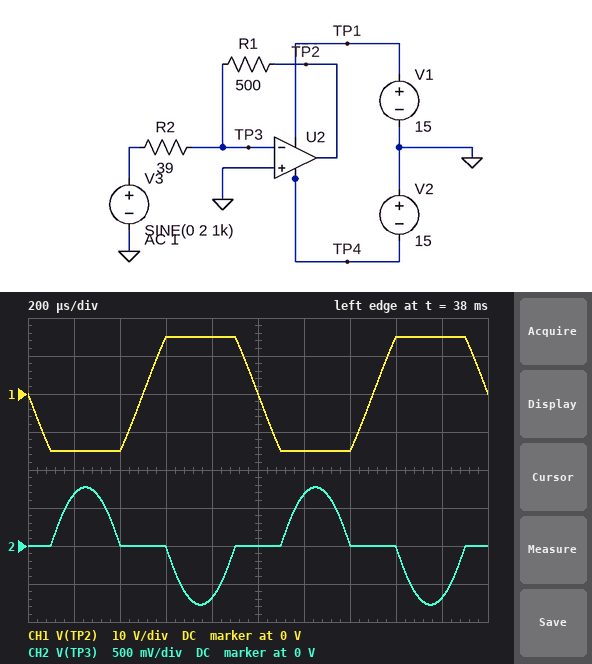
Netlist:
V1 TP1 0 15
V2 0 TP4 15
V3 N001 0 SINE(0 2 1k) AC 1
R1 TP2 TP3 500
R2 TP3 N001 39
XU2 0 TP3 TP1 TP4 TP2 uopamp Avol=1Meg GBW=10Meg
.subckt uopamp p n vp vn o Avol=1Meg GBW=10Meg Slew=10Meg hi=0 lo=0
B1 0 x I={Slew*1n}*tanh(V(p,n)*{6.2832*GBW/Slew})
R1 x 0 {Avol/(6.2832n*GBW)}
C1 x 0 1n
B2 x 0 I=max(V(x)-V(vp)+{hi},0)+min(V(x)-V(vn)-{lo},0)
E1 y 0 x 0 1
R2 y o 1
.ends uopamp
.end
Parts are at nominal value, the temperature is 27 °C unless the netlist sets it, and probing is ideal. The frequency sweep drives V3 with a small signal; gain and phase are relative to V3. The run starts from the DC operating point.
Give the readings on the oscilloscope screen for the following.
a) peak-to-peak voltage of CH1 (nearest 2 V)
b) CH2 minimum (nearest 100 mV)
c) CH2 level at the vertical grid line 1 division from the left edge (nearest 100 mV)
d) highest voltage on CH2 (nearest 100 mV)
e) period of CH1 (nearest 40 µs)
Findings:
30 V
-800 mV
700 mV
800 mV
1.00 ms
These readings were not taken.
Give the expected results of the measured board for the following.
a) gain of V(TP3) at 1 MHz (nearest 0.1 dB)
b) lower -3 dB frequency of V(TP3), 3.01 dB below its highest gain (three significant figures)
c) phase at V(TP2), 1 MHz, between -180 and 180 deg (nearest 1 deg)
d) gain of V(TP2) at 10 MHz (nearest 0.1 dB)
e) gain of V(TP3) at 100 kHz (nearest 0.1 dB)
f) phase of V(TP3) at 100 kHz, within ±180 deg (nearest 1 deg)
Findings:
-2.5 dB
722 kHz
126 deg
-0.7 dB
-17.9 dB
82 deg
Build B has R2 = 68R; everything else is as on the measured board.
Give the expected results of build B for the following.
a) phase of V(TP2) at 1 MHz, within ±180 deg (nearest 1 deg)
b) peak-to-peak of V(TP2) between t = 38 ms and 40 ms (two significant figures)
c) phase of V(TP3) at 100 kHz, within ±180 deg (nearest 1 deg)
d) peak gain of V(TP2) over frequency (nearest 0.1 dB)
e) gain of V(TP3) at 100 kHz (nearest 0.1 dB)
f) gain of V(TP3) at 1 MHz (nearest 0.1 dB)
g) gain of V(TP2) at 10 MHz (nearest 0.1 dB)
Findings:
140 deg
29 V
85 deg
17.3 dB
-22.7 dB
-5.0 dB
-1.2 dB
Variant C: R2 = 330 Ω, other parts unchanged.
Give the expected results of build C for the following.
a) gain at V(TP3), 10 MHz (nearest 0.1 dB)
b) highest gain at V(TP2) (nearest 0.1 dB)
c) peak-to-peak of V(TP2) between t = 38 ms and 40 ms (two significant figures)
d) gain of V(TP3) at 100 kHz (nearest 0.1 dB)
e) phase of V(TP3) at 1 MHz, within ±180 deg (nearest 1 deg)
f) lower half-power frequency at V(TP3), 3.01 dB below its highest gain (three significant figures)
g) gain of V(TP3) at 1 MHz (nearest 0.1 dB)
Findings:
-5.0 dB
3.6 dB
6.1 V
-36.4 dB
76 deg
3.97 MHz
-16.6 dB
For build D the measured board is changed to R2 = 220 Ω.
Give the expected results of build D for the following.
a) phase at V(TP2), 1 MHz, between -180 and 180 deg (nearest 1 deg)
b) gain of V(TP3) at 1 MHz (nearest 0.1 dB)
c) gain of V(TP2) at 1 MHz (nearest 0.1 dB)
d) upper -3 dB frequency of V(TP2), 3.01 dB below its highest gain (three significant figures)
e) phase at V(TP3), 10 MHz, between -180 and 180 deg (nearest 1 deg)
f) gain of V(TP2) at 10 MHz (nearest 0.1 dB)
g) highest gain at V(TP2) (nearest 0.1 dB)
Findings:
162 deg
-13.3 dB
6.7 dB
3.05 MHz
17 deg
-3.6 dB
7.1 dB
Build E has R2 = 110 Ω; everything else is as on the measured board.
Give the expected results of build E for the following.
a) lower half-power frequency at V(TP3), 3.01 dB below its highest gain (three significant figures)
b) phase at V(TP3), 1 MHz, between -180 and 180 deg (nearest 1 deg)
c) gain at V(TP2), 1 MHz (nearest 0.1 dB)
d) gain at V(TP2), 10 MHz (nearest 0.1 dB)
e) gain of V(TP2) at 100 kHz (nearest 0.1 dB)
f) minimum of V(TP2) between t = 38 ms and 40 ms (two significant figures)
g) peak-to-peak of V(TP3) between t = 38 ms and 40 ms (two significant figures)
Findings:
1.80 MHz
61 deg
12.0 dB
-1.9 dB
13.1 dB
-9.1 V
1.8 mV
